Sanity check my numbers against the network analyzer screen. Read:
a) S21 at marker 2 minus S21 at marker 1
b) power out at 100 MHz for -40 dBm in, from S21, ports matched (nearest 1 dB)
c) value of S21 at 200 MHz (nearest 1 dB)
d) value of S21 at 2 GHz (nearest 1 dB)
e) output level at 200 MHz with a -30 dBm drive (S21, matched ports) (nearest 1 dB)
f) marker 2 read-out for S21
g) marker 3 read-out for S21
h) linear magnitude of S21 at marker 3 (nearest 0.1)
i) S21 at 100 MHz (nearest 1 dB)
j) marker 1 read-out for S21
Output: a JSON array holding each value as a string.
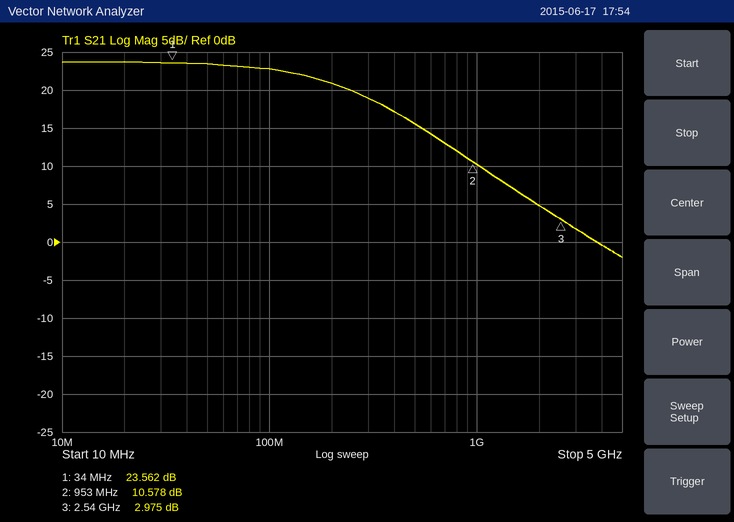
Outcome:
["-12.984 dB", "-17 dBm", "21 dB", "5 dB", "-9 dBm", "10.578 dB", "2.975 dB", "1.4", "23 dB", "23.562 dB"]
